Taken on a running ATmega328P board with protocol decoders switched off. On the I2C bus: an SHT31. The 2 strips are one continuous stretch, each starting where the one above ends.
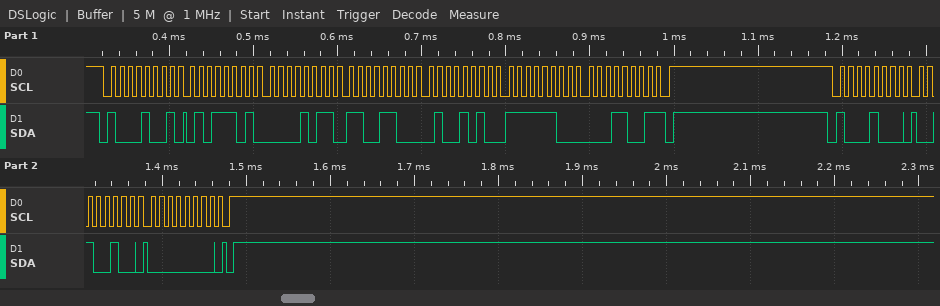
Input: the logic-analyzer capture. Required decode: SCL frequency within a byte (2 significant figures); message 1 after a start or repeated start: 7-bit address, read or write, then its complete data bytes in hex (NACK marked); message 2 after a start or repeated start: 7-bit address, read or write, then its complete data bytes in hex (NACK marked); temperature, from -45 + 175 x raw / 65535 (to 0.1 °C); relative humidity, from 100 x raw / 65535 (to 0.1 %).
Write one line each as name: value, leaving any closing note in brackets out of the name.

SCL frequency within a byte: 100 kHz
message 1 after a start or repeated start: 7-bit address, read or write, then its complete data bytes in hex: 0x44 read: 5D 0B CC 4A FC 19 NACK
message 2 after a start or repeated start: 7-bit address, read or write, then its complete data bytes in hex: 0x44 write: 24 00
temperature, from -45 + 175 x raw / 65535: 18.6 °C
relative humidity, from 100 x raw / 65535: 29.3 %
